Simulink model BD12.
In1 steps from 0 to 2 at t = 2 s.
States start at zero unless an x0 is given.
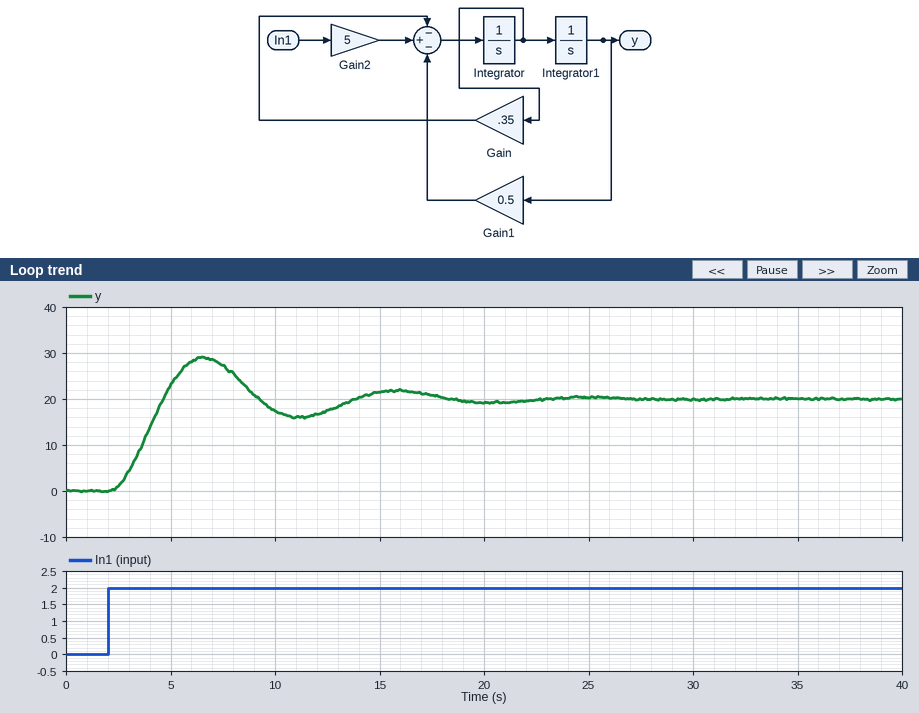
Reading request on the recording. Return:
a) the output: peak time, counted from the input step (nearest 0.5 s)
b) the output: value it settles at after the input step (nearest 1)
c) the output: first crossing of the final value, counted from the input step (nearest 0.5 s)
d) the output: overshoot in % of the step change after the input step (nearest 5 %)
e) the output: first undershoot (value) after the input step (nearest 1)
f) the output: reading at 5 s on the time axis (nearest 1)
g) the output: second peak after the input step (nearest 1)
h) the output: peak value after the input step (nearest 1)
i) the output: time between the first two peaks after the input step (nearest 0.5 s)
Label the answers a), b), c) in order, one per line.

a) 4.5 s
b) 20
c) 2.5 s
d) 45 %
e) 16
f) 23
g) 22
h) 29
i) 9.0 s
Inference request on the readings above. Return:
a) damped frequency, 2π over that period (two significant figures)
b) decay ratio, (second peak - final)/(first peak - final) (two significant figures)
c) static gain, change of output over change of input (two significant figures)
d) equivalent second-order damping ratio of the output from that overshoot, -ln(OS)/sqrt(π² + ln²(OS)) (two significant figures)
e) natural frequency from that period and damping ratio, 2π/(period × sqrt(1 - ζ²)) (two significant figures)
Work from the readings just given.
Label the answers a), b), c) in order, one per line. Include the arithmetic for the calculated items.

a) 2π / 9 = 0.70 rad/s
b) (22 - 20) / (29 - 20) = 0.22
c) (20 - 0) / (2 - 0) = 10
d) ln(0.45) = -0.799; 0.799 / sqrt(9.870 + 0.638) = 0.25
e) 2π / (9 × sqrt(1 - 0.25²)) = 0.72 rad/s
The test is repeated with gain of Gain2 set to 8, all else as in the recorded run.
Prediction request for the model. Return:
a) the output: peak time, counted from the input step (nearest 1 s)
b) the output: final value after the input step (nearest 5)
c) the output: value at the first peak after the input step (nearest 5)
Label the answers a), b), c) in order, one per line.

a) 5 s
b) 30
c) 45
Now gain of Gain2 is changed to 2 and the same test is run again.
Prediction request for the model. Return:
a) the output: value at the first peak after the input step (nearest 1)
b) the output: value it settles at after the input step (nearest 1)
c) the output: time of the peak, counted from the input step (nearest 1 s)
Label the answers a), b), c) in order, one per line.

a) 12
b) 8
c) 5 s
